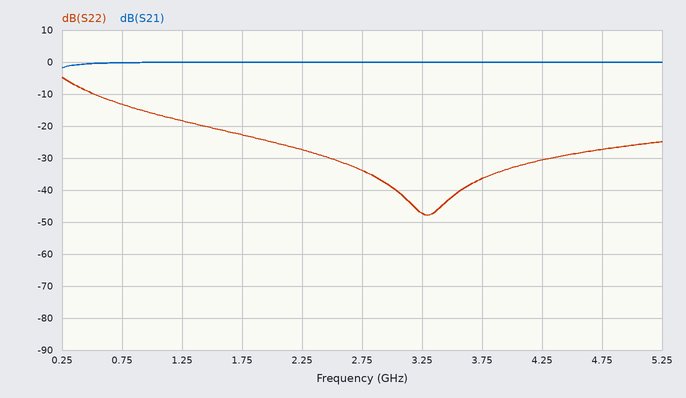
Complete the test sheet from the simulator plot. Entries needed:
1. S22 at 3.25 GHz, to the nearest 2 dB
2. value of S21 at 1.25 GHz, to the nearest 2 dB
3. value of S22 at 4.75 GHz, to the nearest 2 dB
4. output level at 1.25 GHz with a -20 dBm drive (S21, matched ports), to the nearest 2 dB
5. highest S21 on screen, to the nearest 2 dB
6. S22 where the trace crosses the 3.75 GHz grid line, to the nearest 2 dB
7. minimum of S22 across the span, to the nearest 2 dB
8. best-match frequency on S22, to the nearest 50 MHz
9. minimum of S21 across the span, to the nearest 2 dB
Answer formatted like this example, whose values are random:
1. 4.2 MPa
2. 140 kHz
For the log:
1. -48 dB
2. 0 dB
3. -28 dB
4. -20 dBm
5. 0 dB
6. -36 dB
7. -48 dB
8. 3.30 GHz
9. -2 dB
